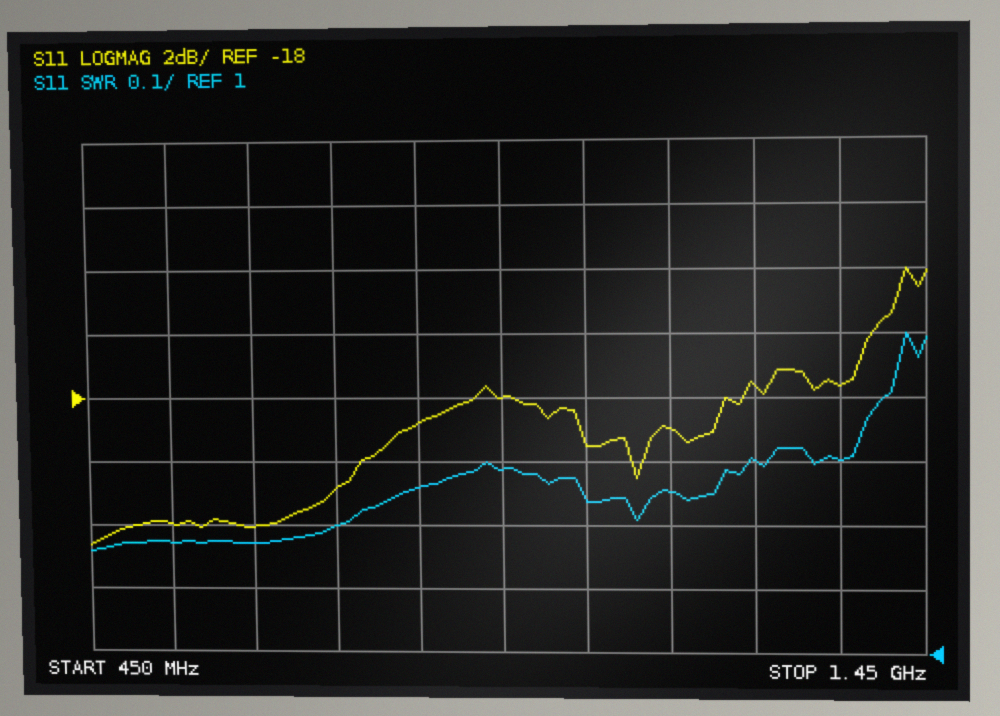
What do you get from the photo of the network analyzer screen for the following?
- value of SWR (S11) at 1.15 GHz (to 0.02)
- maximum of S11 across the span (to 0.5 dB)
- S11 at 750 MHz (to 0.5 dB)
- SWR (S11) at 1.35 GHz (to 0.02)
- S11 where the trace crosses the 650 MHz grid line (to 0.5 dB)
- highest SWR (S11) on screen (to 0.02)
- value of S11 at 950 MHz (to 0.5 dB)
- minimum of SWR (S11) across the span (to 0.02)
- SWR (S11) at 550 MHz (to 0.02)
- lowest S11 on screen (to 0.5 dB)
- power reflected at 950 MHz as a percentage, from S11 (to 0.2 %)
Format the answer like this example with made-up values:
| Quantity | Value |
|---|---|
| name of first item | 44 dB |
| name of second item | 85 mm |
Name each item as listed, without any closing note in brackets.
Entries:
| Quantity | Value |
|---|---|
| value of SWR (S11) at 1.15 GHz | 1.26 |
| maximum of S11 across the span | -14.0 dB |
| S11 at 750 MHz | -21.0 dB |
| SWR (S11) at 1.35 GHz | 1.30 |
| S11 where the trace crosses the 650 MHz grid line | -22.0 dB |
| highest SWR (S11) on screen | 1.50 |
| value of S11 at 950 MHz | -18.0 dB |
| minimum of SWR (S11) across the span | 1.16 |
| SWR (S11) at 550 MHz | 1.18 |
| lowest S11 on screen | -22.5 dB |
| power reflected at 950 MHz as a percentage, from S11 | 1.6 % |
